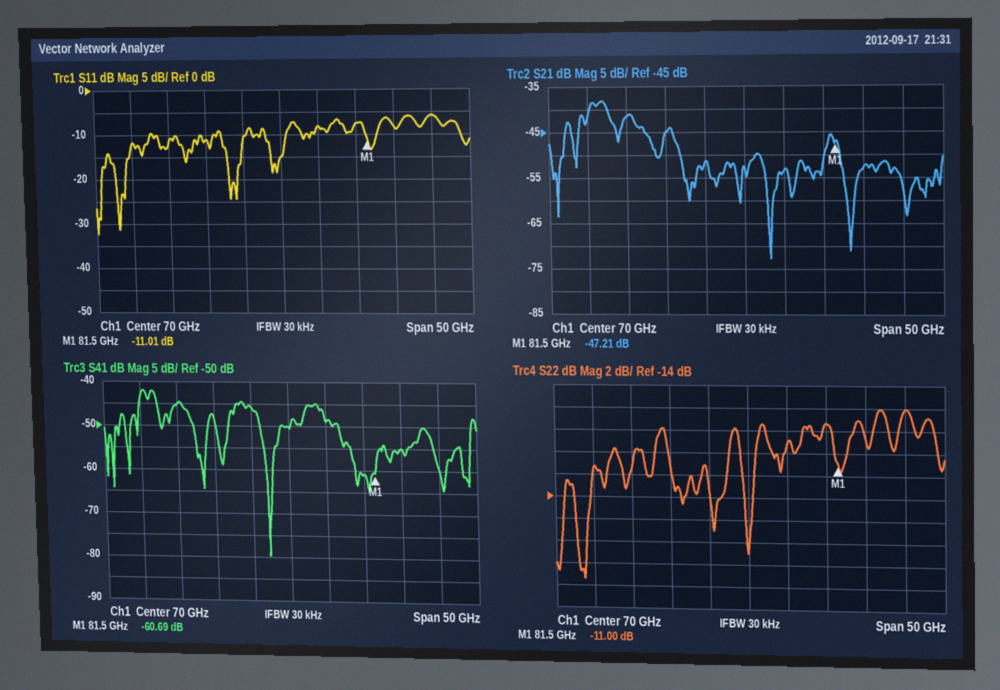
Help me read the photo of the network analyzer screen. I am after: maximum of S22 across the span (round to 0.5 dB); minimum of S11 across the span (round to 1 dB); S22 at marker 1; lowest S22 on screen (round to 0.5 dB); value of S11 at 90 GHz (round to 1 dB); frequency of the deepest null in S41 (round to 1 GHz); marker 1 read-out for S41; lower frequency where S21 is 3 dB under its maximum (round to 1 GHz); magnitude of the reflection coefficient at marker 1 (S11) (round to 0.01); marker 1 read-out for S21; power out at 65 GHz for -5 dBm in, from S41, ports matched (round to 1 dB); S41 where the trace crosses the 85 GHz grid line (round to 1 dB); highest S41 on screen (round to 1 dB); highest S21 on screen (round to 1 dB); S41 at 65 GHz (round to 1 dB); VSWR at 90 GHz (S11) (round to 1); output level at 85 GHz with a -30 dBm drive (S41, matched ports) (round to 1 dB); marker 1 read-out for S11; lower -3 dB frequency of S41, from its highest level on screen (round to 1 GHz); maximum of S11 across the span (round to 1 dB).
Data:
-6.0 dB
-32 dB
-11.00 dB
-21.5 dB
-6 dB
67 GHz
-60.69 dB
50 GHz
0.28
-47.21 dB
-51 dBm
-55 dB
-42 dB
-38 dB
-46 dB
3
-85 dBm
-11.01 dB
50 GHz
-6 dB
